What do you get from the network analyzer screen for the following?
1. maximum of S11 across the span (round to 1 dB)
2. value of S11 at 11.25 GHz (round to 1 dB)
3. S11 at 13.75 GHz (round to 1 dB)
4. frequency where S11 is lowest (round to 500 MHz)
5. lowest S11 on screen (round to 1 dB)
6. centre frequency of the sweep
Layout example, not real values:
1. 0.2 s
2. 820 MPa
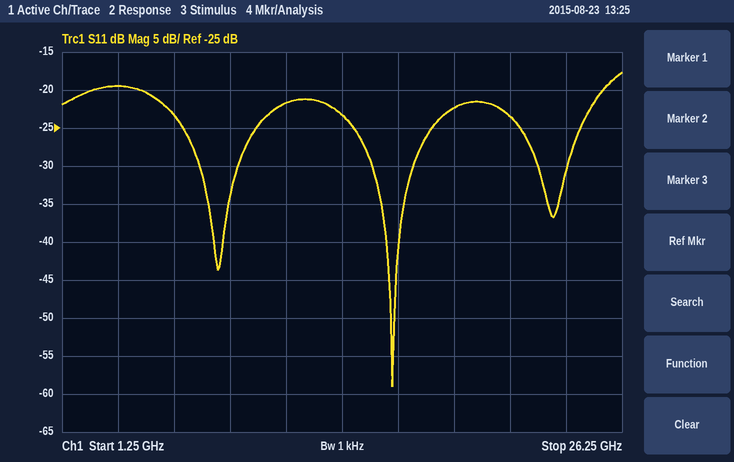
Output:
1. -18 dB
2. -22 dB
3. -23 dB
4. 16.0 GHz
5. -59 dB
6. 13.75 GHz
